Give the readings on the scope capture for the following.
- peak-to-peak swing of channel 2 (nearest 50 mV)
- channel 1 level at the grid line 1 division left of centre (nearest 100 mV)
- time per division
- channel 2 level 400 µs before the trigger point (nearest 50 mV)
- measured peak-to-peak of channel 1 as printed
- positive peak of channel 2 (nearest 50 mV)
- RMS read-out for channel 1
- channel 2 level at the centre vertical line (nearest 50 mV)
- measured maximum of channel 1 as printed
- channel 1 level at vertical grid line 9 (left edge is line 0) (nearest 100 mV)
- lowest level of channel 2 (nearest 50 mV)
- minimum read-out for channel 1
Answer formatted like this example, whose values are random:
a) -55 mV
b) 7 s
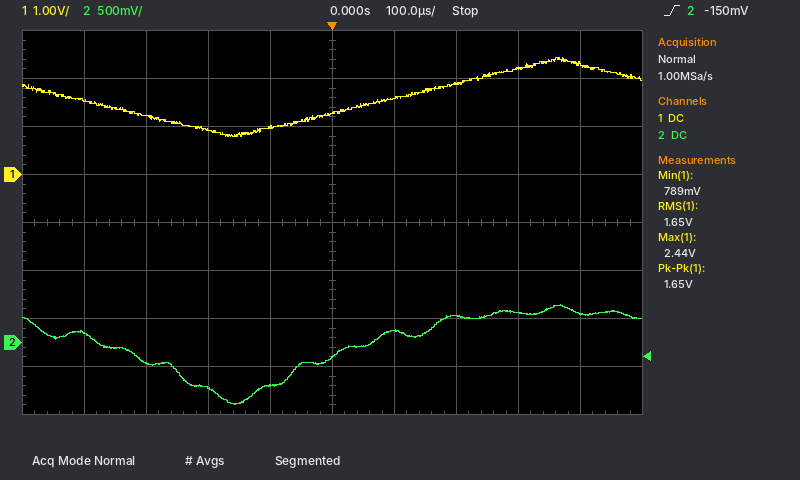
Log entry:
a) 1.05 V
b) 1.0 V
c) 100 µs
d) 100 mV
e) 1.65 V
f) 400 mV
g) 1.65 V
h) -150 mV
i) 2.44 V
j) 2.3 V
k) -650 mV
l) 789 mV
